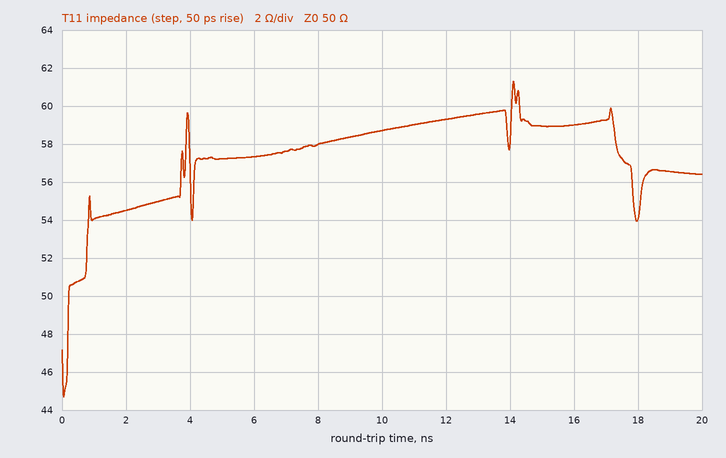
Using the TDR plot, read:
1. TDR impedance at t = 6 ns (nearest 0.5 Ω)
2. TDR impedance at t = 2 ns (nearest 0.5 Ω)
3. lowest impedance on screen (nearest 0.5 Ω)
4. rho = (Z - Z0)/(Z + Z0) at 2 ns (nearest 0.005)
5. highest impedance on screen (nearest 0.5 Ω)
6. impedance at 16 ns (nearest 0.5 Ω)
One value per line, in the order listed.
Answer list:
57.5 Ω
54.5 Ω
44.5 Ω
+0.045
61.5 Ω
59.0 Ω
